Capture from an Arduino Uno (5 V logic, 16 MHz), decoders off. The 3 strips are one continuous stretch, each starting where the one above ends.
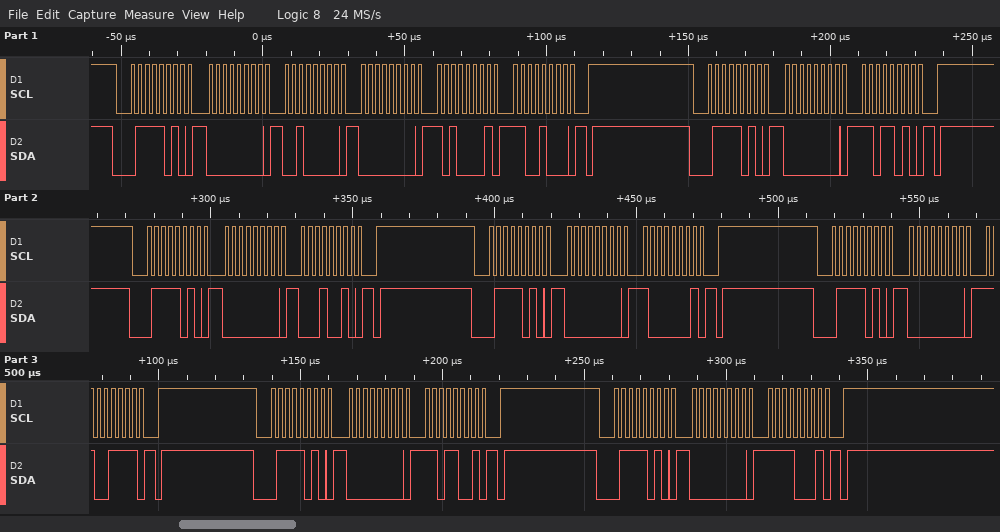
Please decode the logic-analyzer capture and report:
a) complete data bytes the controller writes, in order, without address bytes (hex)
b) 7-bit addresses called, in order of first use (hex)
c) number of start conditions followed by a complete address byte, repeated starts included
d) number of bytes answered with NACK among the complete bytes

00 20 00 A1 C8 00 DA 00 12 00 81 00 CF 00 D9 00 F1
0x3D
7
0
